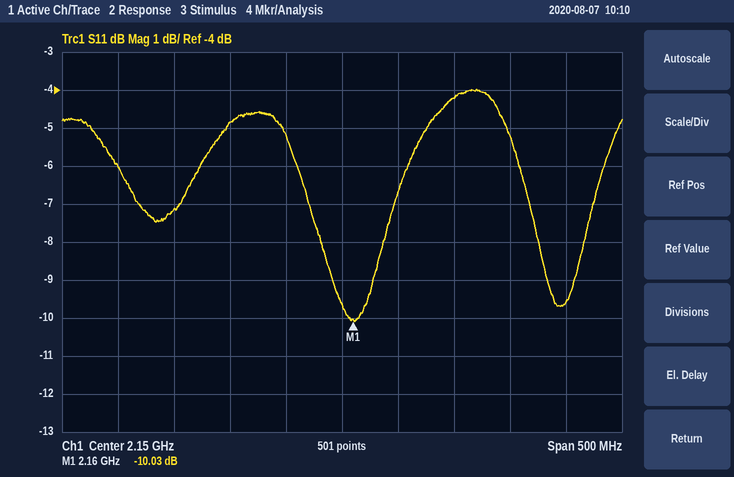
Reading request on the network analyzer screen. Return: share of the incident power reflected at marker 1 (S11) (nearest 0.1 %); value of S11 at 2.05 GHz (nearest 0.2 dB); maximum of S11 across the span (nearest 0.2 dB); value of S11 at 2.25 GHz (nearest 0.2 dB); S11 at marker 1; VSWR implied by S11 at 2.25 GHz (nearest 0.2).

9.9 %
-4.8 dB
-4.0 dB
-4.2 dB
-10.03 dB
4.2
